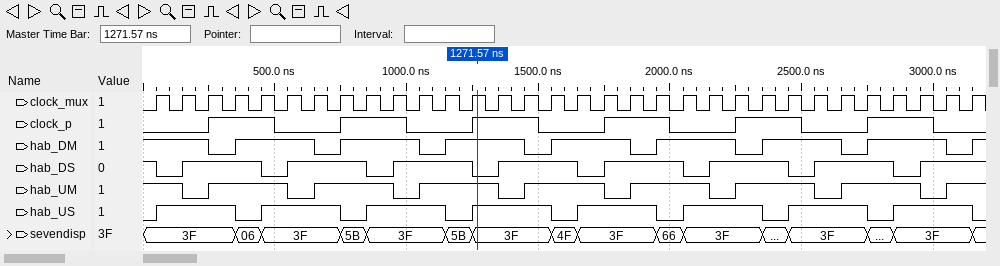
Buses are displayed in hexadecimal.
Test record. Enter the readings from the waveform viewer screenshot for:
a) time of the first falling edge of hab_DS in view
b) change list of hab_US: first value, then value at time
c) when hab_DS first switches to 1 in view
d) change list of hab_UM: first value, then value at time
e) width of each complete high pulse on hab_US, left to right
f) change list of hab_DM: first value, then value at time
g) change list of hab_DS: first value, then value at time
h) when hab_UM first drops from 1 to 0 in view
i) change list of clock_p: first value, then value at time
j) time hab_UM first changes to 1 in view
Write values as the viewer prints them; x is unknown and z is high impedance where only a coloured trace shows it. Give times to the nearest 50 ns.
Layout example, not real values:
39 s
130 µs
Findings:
50 ns
0, 1 at 50 ns, 0 at 350 ns, 1 at 450 ns, 0 at 750 ns, 1 at 850 ns, 0 at 1150 ns, 1 at 1250 ns, 0 at 1550 ns, 1 at 1650 ns, 0 at 1950 ns, 1 at 2050 ns, 0 at 2350 ns, 1 at 2450 ns, 0 at 2750 ns, 1 at 2850 ns, 0 at 3150 ns
150 ns
1, 0 at 150 ns, 1 at 250 ns, 0 at 550 ns, 1 at 650 ns, 0 at 950 ns, 1 at 1050 ns, 0 at 1350 ns, 1 at 1450 ns, 0 at 1750 ns, 1 at 1850 ns, 0 at 2150 ns, 1 at 2250 ns, 0 at 2550 ns, 1 at 2650 ns, 0 at 2950 ns, 1 at 3050 ns
300 ns, 300 ns, 300 ns, 300 ns, 300 ns, 300 ns, 300 ns, 300 ns
1, 0 at 250 ns, 1 at 350 ns, 0 at 650 ns, 1 at 750 ns, 0 at 1050 ns, 1 at 1150 ns, 0 at 1450 ns, 1 at 1550 ns, 0 at 1850 ns, 1 at 1950 ns, 0 at 2250 ns, 1 at 2350 ns, 0 at 2650 ns, 1 at 2750 ns, 0 at 3050 ns, 1 at 3150 ns
1, 0 at 50 ns, 1 at 150 ns, 0 at 450 ns, 1 at 550 ns, 0 at 850 ns, 1 at 950 ns, 0 at 1250 ns, 1 at 1350 ns, 0 at 1650 ns, 1 at 1750 ns, 0 at 2050 ns, 1 at 2150 ns, 0 at 2450 ns, 1 at 2550 ns, 0 at 2850 ns, 1 at 2950 ns
150 ns
0, 1 at 250 ns, 0 at 500 ns, 1 at 750 ns, 0 at 1000 ns, 1 at 1250 ns, 0 at 1500 ns, 1 at 1750 ns, 0 at 2000 ns, 1 at 2250 ns, 0 at 2500 ns, 1 at 2750 ns, 0 at 3000 ns
250 ns
